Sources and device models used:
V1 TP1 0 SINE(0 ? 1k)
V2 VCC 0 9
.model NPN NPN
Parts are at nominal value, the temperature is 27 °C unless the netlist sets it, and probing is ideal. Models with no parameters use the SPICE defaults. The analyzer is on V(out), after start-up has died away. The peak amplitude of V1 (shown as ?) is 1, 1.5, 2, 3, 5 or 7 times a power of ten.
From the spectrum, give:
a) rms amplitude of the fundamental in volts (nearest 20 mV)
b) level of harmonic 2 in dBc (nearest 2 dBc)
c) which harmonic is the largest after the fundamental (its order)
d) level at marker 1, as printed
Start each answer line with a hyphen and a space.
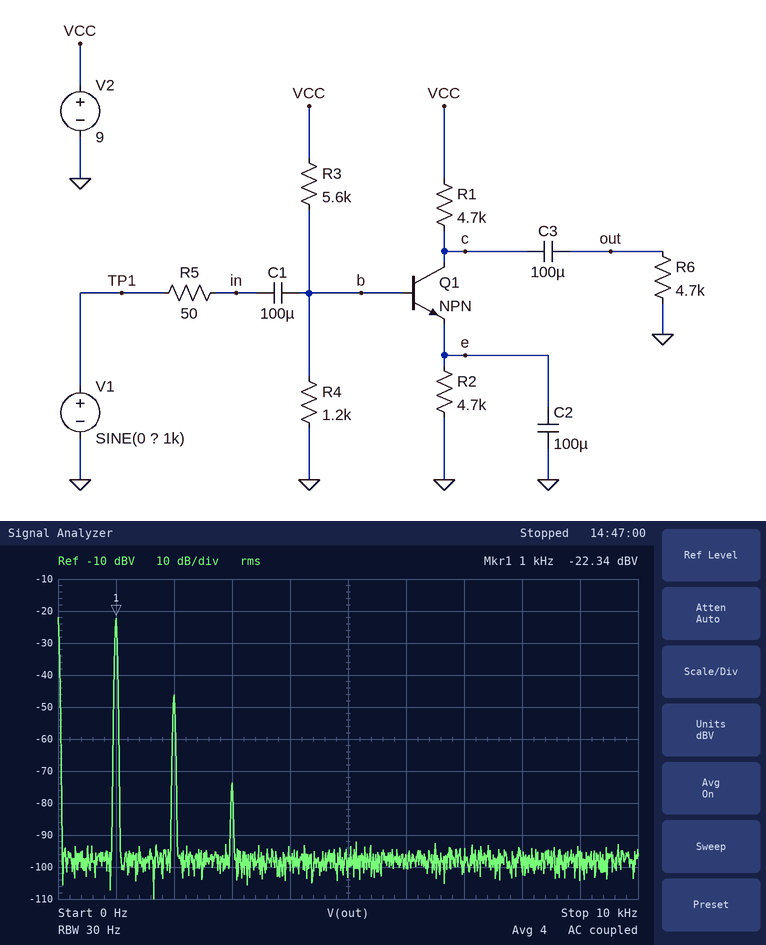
- 80 mV
- -24 dBc
- 2
- -22.34 dBV
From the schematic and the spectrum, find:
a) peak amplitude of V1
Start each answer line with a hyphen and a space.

- 7 mV
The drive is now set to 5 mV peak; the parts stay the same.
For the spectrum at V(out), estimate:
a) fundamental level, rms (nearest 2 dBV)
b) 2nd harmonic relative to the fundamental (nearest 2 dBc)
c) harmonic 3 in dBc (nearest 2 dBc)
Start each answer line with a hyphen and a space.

- -26 dBV
- -26 dBc
- -58 dBc
